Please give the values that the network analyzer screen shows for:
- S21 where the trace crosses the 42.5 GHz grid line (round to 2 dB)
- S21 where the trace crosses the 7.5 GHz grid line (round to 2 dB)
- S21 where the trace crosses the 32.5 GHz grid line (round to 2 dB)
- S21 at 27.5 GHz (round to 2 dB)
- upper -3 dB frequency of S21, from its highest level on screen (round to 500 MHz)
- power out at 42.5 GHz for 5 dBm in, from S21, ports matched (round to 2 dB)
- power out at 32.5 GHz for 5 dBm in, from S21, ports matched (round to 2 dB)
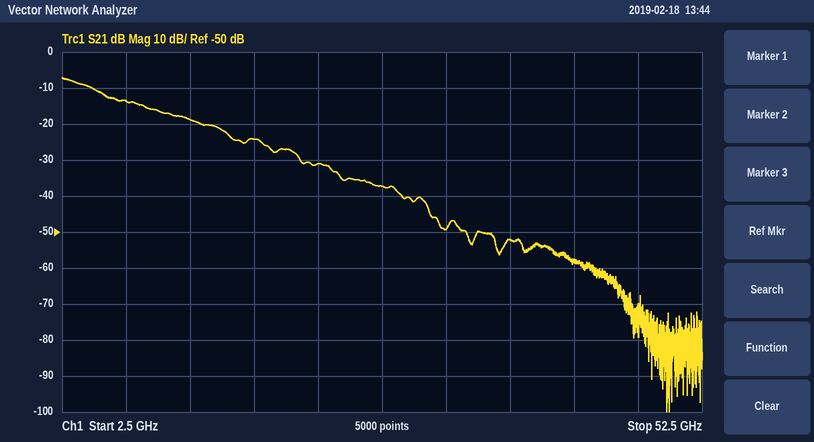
-58 dB
-14 dB
-50 dB
-38 dB
5.0 GHz
-54 dBm
-44 dBm
